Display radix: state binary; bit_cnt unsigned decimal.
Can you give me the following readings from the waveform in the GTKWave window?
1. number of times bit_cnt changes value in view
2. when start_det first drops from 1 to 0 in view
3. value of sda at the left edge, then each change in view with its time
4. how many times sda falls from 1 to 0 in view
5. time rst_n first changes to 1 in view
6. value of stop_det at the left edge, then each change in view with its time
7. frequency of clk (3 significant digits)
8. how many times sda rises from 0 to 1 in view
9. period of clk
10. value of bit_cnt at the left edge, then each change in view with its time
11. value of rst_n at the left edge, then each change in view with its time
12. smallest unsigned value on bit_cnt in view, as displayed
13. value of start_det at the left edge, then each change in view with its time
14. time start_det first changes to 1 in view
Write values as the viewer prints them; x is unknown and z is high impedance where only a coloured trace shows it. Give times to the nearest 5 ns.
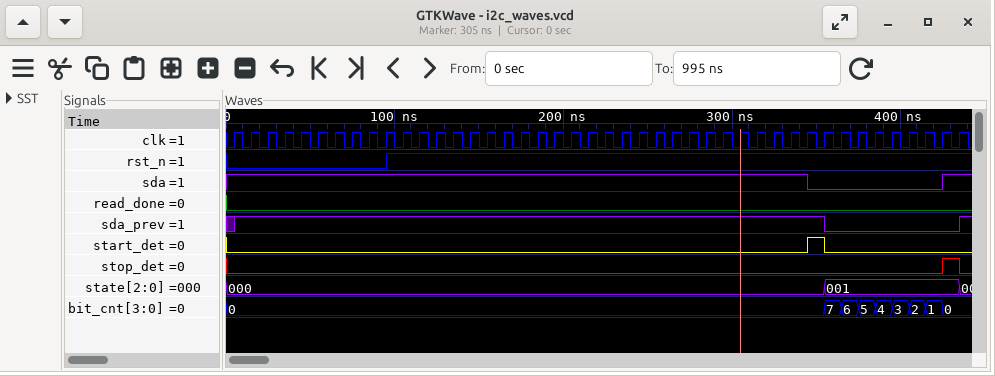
8
355 ns
1, 0 at 345 ns, 1 at 425 ns
1
95 ns
0, 1 at 425 ns, 0 at 435 ns
100 MHz
1
10 ns
0, 7 at 355 ns, 6 at 365 ns, 5 at 375 ns, 4 at 385 ns, 3 at 395 ns, 2 at 405 ns, 1 at 415 ns, 0 at 425 ns
0, 1 at 95 ns
0
0, 1 at 345 ns, 0 at 355 ns
345 ns
